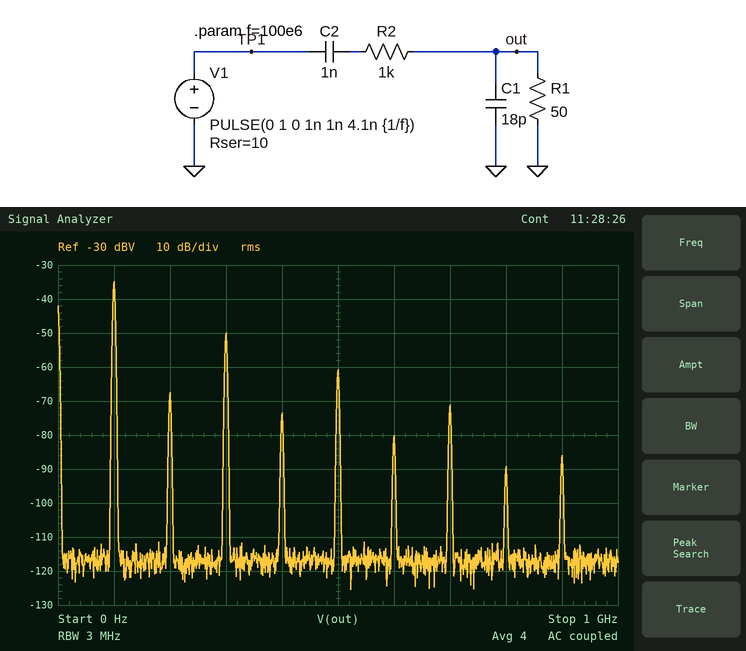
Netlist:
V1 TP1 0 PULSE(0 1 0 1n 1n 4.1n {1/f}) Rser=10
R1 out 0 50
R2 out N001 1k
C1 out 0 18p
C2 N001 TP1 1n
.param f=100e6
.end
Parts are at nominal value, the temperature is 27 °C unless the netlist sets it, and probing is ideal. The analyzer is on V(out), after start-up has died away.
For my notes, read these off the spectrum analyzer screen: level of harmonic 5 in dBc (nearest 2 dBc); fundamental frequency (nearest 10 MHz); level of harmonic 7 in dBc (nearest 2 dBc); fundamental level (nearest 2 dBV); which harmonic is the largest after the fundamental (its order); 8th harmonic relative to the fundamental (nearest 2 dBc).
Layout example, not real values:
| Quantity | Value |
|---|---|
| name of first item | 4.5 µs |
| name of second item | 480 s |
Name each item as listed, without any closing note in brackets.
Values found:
| Quantity | Value |
|---|---|
| level of harmonic 5 in dBc | -26 dBc |
| fundamental frequency | 100 MHz |
| level of harmonic 7 in dBc | -36 dBc |
| fundamental level | -34 dBV |
| which harmonic is the largest after the fundamental | 3 |
| 8th harmonic relative to the fundamental | -54 dBc |
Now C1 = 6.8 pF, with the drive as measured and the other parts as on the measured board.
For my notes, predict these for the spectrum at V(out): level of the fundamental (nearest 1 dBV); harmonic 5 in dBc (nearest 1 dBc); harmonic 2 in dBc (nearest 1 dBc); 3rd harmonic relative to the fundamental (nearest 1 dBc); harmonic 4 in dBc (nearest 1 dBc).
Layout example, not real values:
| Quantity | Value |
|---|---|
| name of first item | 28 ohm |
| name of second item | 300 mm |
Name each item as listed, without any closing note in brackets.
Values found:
| Quantity | Value |
|---|---|
| level of the fundamental | -34 dBV |
| harmonic 5 in dBc | -21 dBc |
| harmonic 2 in dBc | -31 dBc |
| 3rd harmonic relative to the fundamental | -12 dBc |
| harmonic 4 in dBc | -34 dBc |
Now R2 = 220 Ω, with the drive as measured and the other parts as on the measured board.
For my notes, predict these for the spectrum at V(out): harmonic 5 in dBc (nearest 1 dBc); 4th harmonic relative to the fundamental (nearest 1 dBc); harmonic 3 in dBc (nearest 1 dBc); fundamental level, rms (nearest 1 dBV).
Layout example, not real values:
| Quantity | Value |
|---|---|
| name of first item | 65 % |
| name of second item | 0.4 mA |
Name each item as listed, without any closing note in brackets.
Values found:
| Quantity | Value |
|---|---|
| harmonic 5 in dBc | -25 dBc |
| 4th harmonic relative to the fundamental | -38 dBc |
| harmonic 3 in dBc | -15 dBc |
| fundamental level, rms | -23 dBV |
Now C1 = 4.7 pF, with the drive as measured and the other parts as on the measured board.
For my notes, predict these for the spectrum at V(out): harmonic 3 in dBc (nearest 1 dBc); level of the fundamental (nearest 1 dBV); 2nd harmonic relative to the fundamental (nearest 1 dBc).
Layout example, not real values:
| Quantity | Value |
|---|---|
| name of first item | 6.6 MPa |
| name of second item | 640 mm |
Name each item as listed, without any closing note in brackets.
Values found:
| Quantity | Value |
|---|---|
| harmonic 3 in dBc | -11 dBc |
| level of the fundamental | -34 dBV |
| 2nd harmonic relative to the fundamental | -31 dBc |
